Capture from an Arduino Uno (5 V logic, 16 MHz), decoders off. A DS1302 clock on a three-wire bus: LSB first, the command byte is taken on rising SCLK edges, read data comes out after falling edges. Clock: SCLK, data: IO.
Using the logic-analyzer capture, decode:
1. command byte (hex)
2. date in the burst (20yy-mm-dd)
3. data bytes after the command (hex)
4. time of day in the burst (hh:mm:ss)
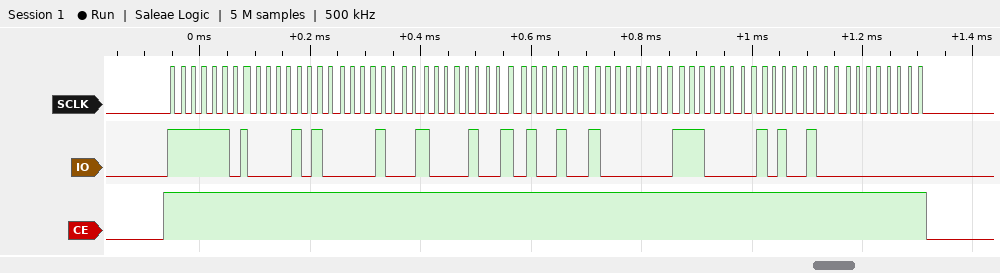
0xBF
2025-01-25
50 10 21 25 01 07 25 00
21:10:50
